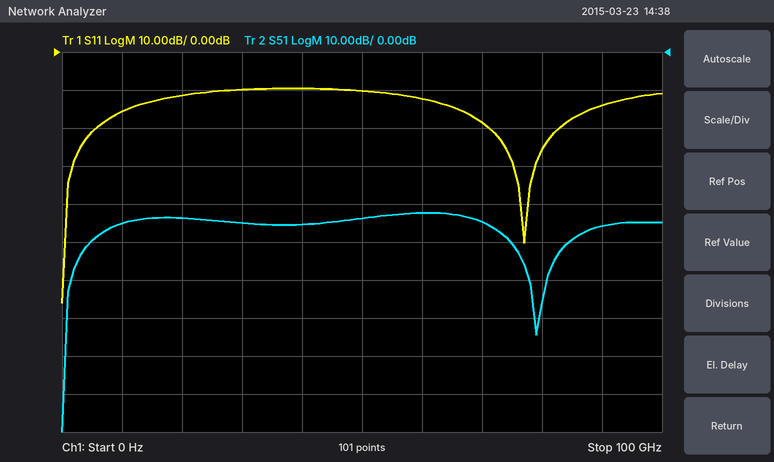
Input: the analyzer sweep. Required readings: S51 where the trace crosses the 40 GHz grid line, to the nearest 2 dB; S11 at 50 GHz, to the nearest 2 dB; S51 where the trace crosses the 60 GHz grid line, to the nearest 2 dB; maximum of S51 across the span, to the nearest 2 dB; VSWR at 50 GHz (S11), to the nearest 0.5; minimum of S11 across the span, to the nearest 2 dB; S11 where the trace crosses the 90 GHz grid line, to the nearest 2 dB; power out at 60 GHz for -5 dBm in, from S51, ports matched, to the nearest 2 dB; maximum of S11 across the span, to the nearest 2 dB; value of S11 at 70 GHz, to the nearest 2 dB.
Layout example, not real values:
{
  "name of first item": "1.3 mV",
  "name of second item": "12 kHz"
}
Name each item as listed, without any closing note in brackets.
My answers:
{
  "S51 where the trace crosses the 40 GHz grid line, to the nearest 2 dB": "-46 dB",
  "S11 at 50 GHz, to the nearest 2 dB": "-10 dB",
  "S51 where the trace crosses the 60 GHz grid line, to the nearest 2 dB": "-42 dB",
  "maximum of S51 across the span, to the nearest 2 dB": "-42 dB",
  "VSWR at 50 GHz (S11), to the nearest 0.5": "2.0",
  "minimum of S11 across the span, to the nearest 2 dB": "-66 dB",
  "S11 where the trace crosses the 90 GHz grid line, to the nearest 2 dB": "-14 dB",
  "power out at 60 GHz for -5 dBm in, from S51, ports matched, to the nearest 2 dB": "-48 dBm",
  "maximum of S11 across the span, to the nearest 2 dB": "-10 dB",
  "value of S11 at 70 GHz, to the nearest 2 dB": "-18 dB"
}
